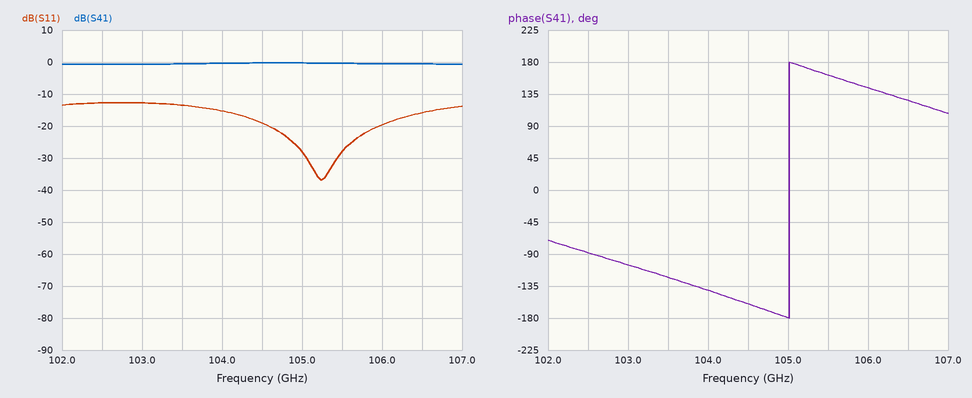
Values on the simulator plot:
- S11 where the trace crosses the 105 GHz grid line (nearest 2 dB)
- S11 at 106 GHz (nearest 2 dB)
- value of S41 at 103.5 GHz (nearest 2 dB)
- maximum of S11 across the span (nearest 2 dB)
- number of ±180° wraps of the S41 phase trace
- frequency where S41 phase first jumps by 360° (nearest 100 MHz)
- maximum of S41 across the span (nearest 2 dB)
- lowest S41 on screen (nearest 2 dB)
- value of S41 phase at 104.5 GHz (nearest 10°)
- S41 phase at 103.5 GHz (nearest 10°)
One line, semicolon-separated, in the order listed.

-28 dB; -20 dB; 0 dB; -12 dB; 1; 105.0 GHz; 0 dB; 0 dB; -160°; -120°
